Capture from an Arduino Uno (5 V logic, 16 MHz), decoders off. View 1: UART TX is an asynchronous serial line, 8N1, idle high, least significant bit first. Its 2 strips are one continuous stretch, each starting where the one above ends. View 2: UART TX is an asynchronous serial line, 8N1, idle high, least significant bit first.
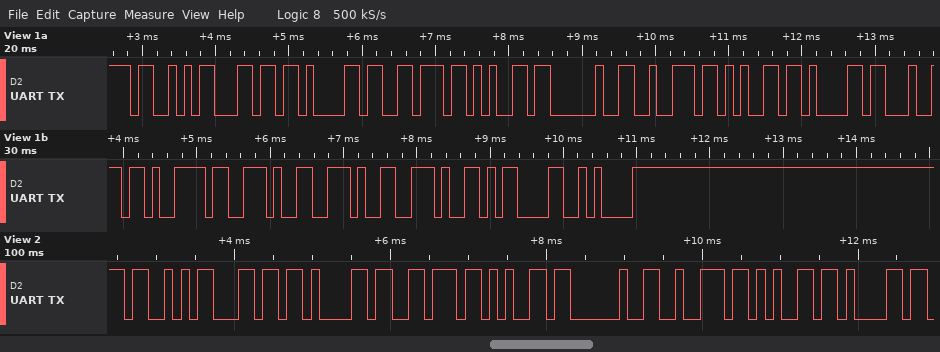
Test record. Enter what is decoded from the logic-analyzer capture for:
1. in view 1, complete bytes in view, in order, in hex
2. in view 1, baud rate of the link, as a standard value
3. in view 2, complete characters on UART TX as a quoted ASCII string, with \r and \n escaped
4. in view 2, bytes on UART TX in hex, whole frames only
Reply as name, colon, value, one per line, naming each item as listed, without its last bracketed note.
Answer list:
in view 1, complete bytes in view, in order, in hex: 53 6C 61 76 65 20 72 65 61 64 79 2E 2E 2E 0D 0A
in view 1, baud rate of the link, as a standard value: 9600 baud
in view 2, complete characters on UART TX as a quoted ASCII string, with \r and \n escaped: "Slave rea"
in view 2, bytes on UART TX in hex, whole frames only: 53 6C 61 76 65 20 72 65 61
